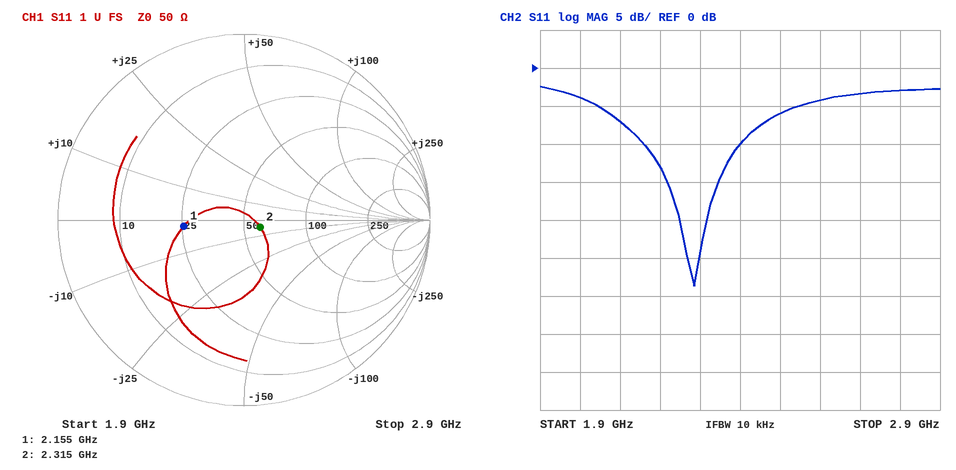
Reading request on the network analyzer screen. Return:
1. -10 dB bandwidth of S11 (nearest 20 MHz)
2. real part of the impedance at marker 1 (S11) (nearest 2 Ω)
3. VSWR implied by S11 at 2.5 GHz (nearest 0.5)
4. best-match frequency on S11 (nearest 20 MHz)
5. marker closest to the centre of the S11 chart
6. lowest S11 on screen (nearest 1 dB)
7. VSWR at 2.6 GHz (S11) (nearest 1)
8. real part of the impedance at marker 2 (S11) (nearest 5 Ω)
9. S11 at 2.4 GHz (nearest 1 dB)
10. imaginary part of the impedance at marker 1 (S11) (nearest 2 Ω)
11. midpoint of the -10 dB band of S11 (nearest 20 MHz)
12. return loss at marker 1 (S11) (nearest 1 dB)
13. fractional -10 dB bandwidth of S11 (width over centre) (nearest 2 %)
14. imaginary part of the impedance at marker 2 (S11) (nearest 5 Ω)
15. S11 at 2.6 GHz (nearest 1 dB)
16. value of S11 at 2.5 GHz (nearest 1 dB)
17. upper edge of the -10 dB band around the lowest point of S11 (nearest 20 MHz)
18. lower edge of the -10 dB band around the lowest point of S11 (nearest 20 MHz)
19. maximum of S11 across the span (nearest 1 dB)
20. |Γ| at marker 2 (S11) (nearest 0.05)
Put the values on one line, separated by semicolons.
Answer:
240 MHz; 26 Ω; 3.0; 2.28 GHz; marker 2; -29 dB; 4; 60 Ω; -10 dB; -2 Ω; 2.28 GHz; 10 dB; 10 %; -5 Ω; -4 dB; -6 dB; 2.40 GHz; 2.16 GHz; -2 dB; 0.10
